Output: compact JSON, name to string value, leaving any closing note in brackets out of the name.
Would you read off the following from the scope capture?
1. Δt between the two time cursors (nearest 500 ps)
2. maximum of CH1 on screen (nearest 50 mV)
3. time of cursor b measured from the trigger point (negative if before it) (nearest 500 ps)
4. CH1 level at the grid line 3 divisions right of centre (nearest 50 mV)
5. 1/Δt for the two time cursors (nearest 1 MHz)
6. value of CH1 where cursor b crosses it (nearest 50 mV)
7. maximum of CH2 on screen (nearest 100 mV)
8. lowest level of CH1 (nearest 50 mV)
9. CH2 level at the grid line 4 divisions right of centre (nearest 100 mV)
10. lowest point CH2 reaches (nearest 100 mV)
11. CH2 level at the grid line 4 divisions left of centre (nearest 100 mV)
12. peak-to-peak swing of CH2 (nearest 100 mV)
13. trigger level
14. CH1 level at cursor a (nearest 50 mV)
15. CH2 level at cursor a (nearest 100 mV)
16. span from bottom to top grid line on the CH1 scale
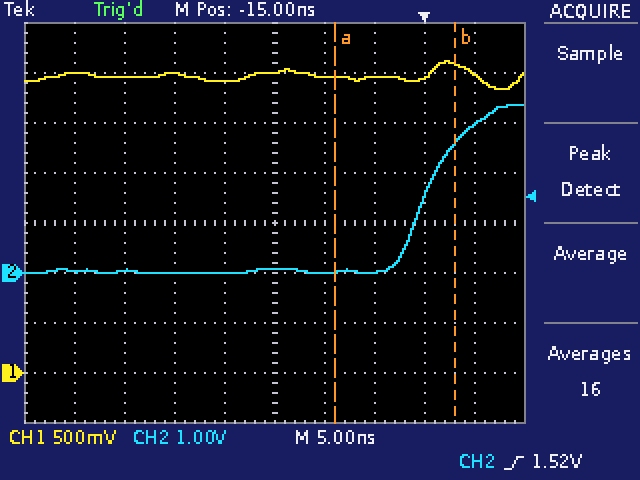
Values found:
{"Δt between the two time cursors": "12.0 ns", "maximum of CH1 on screen": "3.10 V", "time of cursor b measured from the trigger point (negative if before it)": "+3.0 ns", "CH1 level at the grid line 3 divisions right of centre": "2.95 V", "1/Δt for the two time cursors": "83 MHz", "value of CH1 where cursor b crosses it": "3.10 V", "maximum of CH2 on screen": "3.4 V", "lowest level of CH1": "2.85 V", "CH2 level at the grid line 4 divisions right of centre": "3.0 V", "lowest point CH2 reaches": "0.0 V", "CH2 level at the grid line 4 divisions left of centre": "0.0 V", "peak-to-peak swing of CH2": "3.4 V", "trigger level": "1.52 V", "CH1 level at cursor a": "2.95 V", "CH2 level at cursor a": "0.0 V", "span from bottom to top grid line on the CH1 scale": "4 V"}
